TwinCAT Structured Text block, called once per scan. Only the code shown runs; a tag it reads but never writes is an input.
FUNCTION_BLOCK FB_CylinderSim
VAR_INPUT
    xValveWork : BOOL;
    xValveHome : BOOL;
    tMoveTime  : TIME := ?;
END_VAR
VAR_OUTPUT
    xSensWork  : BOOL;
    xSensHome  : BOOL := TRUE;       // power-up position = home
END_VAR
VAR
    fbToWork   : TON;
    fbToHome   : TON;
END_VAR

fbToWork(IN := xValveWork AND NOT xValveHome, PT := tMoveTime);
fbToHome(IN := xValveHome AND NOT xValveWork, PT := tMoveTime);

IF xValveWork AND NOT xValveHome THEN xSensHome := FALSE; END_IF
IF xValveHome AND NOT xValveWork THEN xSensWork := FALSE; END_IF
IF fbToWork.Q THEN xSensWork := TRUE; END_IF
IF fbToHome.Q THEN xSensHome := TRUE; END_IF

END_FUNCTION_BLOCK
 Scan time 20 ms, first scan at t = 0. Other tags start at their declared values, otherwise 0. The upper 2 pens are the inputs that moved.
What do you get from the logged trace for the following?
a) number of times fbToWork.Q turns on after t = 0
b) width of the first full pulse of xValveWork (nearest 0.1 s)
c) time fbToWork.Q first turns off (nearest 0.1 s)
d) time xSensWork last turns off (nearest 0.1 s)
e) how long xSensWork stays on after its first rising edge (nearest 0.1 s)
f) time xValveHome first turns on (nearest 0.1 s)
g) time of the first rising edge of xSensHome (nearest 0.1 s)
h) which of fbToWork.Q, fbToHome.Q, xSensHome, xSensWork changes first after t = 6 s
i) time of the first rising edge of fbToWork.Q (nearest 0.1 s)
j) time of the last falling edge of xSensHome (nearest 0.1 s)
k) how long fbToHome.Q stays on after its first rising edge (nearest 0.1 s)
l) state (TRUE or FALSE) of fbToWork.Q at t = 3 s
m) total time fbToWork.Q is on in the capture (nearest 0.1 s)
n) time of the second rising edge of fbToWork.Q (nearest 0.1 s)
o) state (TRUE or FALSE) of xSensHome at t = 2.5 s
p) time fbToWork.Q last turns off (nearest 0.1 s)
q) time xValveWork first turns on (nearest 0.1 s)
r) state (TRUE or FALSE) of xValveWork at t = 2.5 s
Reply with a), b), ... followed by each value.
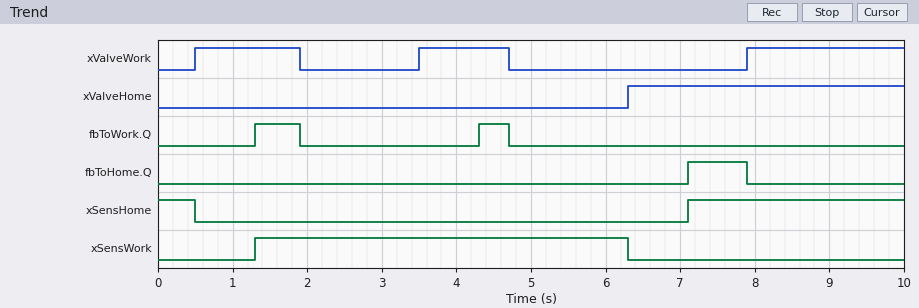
a) 2
b) 1.4 s
c) 1.9 s
d) 6.3 s
e) 5.0 s
f) 6.3 s
g) 7.1 s
h) xSensWork
i) 1.3 s
j) 0.5 s
k) 0.8 s
l) FALSE
m) 1.0 s
n) 4.3 s
o) FALSE
p) 4.7 s
q) 0.5 s
r) FALSE
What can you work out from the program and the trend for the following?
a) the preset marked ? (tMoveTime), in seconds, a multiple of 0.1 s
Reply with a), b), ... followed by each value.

a) 0.8 s
